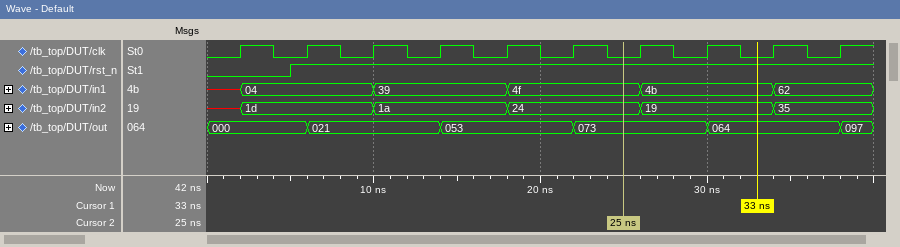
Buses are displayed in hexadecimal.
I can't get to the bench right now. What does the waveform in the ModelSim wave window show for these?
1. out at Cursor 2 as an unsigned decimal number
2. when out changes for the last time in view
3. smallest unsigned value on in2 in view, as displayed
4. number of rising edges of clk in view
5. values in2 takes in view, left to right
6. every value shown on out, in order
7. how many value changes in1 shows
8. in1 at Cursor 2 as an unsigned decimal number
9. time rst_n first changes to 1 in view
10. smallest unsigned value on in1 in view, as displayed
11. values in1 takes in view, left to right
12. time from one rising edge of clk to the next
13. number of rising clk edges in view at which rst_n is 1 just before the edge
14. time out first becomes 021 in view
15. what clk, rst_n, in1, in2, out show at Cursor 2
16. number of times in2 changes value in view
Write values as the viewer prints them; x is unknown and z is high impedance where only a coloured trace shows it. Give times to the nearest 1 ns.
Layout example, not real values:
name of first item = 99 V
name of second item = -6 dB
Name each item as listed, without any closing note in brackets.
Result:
out at Cursor 2 as an unsigned decimal number = 115
when out changes for the last time in view = 38 ns
smallest unsigned value on in2 in view, as displayed = 19
number of rising edges of clk in view = 10
values in2 takes in view, left to right = x, 1d, 1a, 24, 19, 35
every value shown on out, in order = 000, 021, 053, 073, 064, 097
how many value changes in1 shows = 5
in1 at Cursor 2 as an unsigned decimal number = 79
time rst_n first changes to 1 in view = 5 ns
smallest unsigned value on in1 in view, as displayed = 04
values in1 takes in view, left to right = x, 04, 39, 4f, 4b, 62
time from one rising edge of clk to the next = 4 ns
number of rising clk edges in view at which rst_n is 1 just before the edge = 9
time out first becomes 021 in view = 6 ns
what clk, rst_n, in1, in2, out show at Cursor 2 = clk=0, rst_n=1, in1=4f, in2=24, out=073
number of times in2 changes value in view = 5
